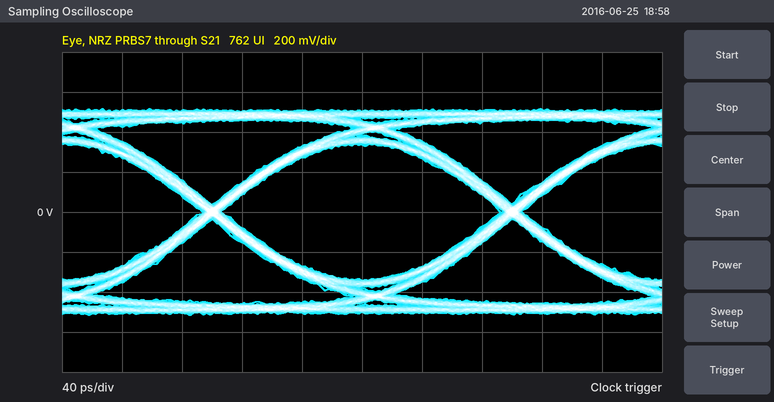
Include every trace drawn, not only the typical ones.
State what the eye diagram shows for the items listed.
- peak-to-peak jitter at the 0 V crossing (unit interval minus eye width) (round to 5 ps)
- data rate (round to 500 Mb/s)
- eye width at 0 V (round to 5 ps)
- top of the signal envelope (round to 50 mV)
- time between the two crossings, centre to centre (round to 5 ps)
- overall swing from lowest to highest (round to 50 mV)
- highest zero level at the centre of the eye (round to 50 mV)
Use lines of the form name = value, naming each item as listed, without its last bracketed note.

peak-to-peak jitter at the 0 V crossing (unit interval minus eye width) = 15 ps
data rate = 5.0 Gb/s
eye width at 0 V = 185 ps
top of the signal envelope = 500 mV
time between the two crossings, centre to centre = 200 ps
overall swing from lowest to highest = 1.05 V
highest zero level at the centre of the eye = -350 mV
